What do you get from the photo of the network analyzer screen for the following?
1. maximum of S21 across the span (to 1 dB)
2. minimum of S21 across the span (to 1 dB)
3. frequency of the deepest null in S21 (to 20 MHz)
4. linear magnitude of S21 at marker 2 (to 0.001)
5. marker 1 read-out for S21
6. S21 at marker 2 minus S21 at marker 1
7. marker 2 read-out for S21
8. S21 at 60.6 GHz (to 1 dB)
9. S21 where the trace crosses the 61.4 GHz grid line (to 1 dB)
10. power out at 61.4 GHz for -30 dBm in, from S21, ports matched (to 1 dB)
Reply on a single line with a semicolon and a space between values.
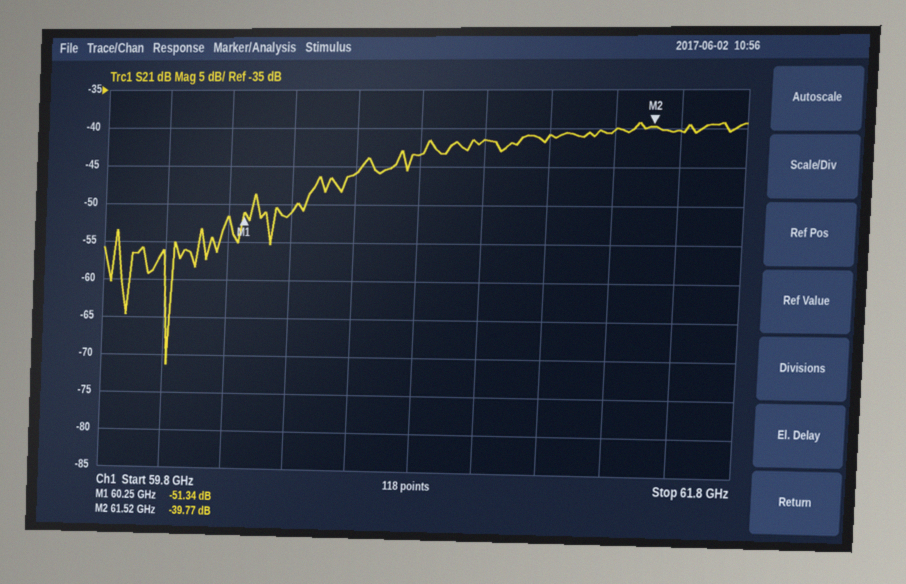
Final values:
-39 dB; -71 dB; 60.02 GHz; 0.010; -51.34 dB; 11.57 dB; -39.77 dB; -46 dB; -40 dB; -70 dBm
